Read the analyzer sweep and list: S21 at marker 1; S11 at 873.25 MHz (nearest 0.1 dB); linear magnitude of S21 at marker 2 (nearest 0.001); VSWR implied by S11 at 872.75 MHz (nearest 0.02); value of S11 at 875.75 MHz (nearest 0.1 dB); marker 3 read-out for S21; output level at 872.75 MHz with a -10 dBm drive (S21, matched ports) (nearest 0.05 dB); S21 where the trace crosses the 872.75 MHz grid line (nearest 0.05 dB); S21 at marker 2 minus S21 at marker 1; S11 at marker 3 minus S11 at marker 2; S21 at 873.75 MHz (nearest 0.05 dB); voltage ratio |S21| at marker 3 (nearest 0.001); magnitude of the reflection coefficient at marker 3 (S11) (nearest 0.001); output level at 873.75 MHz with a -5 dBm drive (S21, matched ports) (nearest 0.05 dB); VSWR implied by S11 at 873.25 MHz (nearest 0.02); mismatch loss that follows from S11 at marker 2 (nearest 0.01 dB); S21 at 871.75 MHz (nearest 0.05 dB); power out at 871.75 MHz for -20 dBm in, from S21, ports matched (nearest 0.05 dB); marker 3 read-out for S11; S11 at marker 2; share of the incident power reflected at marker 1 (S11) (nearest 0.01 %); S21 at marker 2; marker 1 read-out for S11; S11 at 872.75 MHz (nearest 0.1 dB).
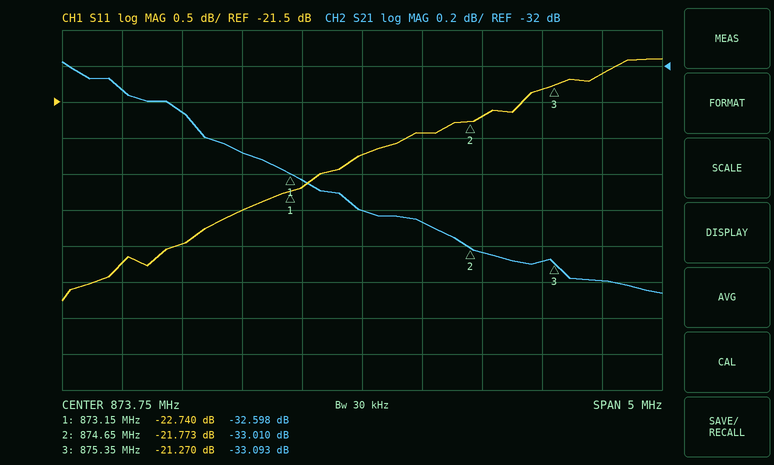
-32.598 dB
-22.7 dB
0.022
1.16
-21.1 dB
-33.093 dB
-42.50 dBm
-32.50 dB
-0.412 dB
0.503 dB
-32.80 dB
0.022
0.086
-37.80 dBm
1.16
0.03 dB
-32.15 dB
-52.15 dBm
-21.270 dB
-21.773 dB
0.53 %
-33.010 dB
-22.740 dB
-23.0 dB
